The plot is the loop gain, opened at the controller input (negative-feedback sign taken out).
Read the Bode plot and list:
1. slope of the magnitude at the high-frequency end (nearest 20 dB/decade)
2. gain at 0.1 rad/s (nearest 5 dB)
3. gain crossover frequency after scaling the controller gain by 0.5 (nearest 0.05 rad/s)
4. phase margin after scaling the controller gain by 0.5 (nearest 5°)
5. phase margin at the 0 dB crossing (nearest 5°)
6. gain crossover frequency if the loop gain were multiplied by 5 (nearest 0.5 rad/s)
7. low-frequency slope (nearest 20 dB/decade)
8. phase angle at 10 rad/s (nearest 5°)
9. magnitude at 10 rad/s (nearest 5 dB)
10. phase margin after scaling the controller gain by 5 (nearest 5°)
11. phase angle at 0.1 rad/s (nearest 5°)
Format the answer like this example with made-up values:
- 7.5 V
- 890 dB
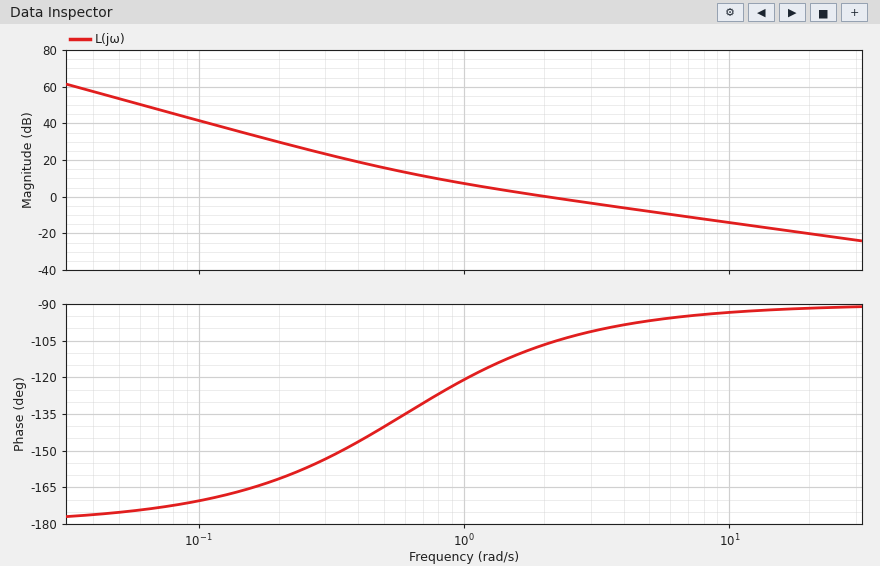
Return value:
- -20 dB/decade
- 40 dB
- 1.10 rad/s
- 60°
- 75°
- 10.0 rad/s
- -40 dB/decade
- -95°
- -15 dB
- 85°
- -170°
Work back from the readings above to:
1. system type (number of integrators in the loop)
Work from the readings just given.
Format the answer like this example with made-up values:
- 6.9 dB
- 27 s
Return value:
- 2
